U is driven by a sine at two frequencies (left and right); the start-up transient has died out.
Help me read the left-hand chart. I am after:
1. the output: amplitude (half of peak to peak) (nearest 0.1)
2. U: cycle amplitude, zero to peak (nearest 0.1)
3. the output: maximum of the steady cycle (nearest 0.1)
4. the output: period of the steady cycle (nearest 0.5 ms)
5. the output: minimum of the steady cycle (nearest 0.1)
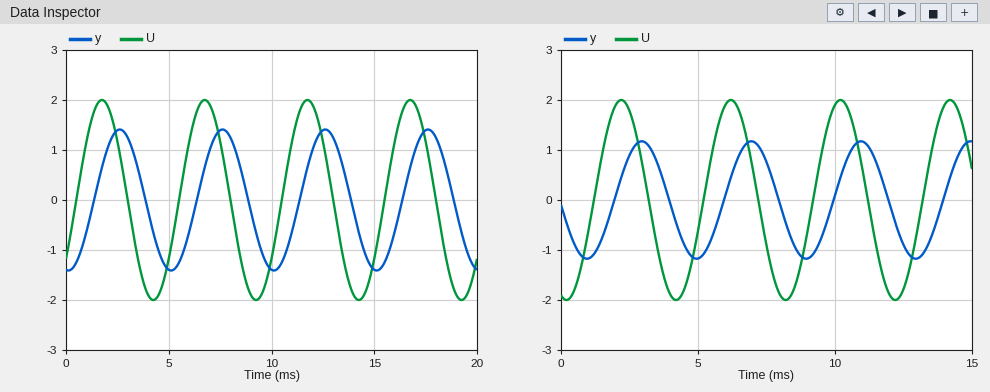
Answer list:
1.4
2.0
1.4
5.0 ms
-1.4
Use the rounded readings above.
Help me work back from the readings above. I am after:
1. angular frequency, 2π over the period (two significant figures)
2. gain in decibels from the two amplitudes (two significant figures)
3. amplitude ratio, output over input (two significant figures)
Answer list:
1.3 rad/ms
-3.1 dB
0.70
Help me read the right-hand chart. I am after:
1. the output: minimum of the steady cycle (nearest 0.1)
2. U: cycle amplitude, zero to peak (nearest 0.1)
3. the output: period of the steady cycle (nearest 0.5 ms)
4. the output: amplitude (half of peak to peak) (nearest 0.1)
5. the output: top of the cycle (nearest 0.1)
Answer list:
-1.2
2.0
4.0 ms
1.2
1.2
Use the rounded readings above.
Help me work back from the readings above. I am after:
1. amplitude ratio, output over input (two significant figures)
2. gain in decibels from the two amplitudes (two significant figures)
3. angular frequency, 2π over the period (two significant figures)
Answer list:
0.60
-4.4 dB
1.6 rad/ms
